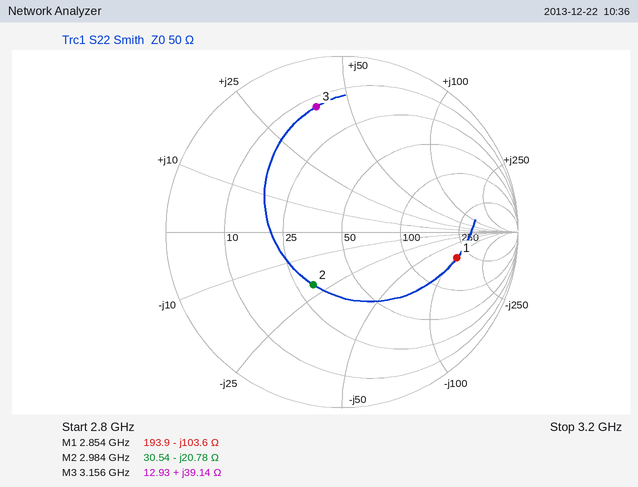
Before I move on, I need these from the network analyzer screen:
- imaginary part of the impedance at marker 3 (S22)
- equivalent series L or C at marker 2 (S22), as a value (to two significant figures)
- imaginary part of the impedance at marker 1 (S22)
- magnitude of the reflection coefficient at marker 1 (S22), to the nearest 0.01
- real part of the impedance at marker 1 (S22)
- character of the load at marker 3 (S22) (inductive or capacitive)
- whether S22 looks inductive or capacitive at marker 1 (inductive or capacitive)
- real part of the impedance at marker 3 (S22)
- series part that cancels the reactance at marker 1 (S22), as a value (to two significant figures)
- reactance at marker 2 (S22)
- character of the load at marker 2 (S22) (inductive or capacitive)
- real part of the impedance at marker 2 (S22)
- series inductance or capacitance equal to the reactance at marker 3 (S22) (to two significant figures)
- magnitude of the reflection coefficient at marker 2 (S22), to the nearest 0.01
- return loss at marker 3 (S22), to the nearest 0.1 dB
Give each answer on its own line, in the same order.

+39.14 Ω
2.6 pF
-103.6 Ω
0.67
193.9 Ω
inductive
capacitive
12.93 Ω
5.8 nH
-20.78 Ω
capacitive
30.54 Ω
2.0 nH
0.34
2.8 dB
